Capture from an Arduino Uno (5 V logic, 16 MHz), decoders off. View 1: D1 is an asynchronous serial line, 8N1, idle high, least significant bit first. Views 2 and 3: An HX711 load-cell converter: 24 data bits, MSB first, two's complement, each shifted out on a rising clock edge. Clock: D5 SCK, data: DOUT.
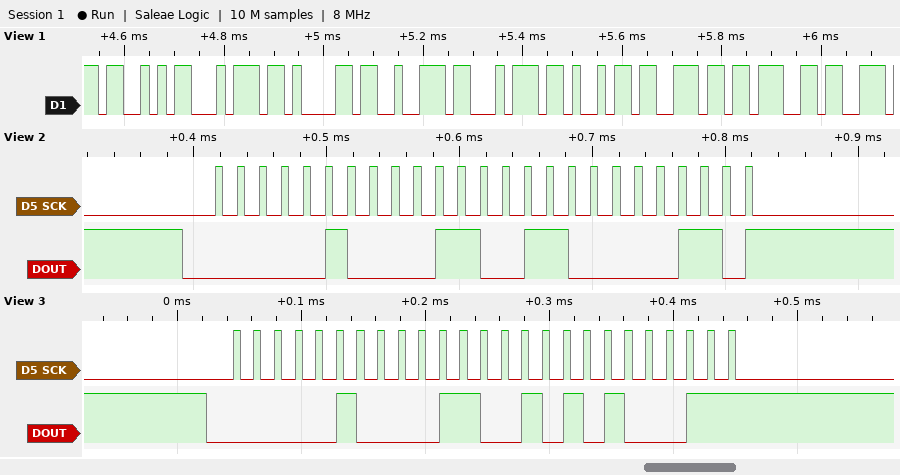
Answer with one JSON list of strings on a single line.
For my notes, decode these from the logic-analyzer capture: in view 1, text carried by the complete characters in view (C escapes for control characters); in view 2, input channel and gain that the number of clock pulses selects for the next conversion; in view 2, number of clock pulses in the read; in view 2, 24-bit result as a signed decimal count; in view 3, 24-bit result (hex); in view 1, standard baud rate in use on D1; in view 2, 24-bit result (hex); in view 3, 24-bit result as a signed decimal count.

["\"Starting\"", "channel A, gain 128", "25", "275206", "0x0432A3", "57600 baud", "0x043306", "275107"]
